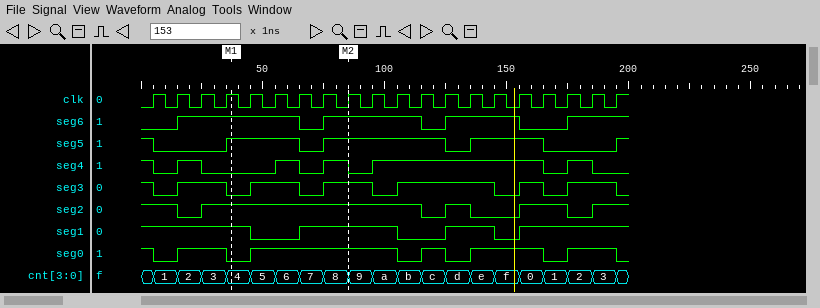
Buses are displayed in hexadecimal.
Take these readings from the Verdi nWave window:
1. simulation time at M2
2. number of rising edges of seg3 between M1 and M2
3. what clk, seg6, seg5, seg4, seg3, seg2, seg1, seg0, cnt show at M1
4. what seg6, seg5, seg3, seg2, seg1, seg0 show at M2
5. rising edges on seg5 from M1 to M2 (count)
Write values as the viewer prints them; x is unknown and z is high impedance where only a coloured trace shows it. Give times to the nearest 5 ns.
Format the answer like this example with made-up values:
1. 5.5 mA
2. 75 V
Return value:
1. 85 ns
2. 2
3. clk=1, seg6=1, seg5=1, seg4=0, seg3=0, seg2=1, seg1=1, seg0=0, cnt=4
4. seg6=1, seg5=1, seg3=1, seg2=1, seg1=1, seg0=1
5. 1
